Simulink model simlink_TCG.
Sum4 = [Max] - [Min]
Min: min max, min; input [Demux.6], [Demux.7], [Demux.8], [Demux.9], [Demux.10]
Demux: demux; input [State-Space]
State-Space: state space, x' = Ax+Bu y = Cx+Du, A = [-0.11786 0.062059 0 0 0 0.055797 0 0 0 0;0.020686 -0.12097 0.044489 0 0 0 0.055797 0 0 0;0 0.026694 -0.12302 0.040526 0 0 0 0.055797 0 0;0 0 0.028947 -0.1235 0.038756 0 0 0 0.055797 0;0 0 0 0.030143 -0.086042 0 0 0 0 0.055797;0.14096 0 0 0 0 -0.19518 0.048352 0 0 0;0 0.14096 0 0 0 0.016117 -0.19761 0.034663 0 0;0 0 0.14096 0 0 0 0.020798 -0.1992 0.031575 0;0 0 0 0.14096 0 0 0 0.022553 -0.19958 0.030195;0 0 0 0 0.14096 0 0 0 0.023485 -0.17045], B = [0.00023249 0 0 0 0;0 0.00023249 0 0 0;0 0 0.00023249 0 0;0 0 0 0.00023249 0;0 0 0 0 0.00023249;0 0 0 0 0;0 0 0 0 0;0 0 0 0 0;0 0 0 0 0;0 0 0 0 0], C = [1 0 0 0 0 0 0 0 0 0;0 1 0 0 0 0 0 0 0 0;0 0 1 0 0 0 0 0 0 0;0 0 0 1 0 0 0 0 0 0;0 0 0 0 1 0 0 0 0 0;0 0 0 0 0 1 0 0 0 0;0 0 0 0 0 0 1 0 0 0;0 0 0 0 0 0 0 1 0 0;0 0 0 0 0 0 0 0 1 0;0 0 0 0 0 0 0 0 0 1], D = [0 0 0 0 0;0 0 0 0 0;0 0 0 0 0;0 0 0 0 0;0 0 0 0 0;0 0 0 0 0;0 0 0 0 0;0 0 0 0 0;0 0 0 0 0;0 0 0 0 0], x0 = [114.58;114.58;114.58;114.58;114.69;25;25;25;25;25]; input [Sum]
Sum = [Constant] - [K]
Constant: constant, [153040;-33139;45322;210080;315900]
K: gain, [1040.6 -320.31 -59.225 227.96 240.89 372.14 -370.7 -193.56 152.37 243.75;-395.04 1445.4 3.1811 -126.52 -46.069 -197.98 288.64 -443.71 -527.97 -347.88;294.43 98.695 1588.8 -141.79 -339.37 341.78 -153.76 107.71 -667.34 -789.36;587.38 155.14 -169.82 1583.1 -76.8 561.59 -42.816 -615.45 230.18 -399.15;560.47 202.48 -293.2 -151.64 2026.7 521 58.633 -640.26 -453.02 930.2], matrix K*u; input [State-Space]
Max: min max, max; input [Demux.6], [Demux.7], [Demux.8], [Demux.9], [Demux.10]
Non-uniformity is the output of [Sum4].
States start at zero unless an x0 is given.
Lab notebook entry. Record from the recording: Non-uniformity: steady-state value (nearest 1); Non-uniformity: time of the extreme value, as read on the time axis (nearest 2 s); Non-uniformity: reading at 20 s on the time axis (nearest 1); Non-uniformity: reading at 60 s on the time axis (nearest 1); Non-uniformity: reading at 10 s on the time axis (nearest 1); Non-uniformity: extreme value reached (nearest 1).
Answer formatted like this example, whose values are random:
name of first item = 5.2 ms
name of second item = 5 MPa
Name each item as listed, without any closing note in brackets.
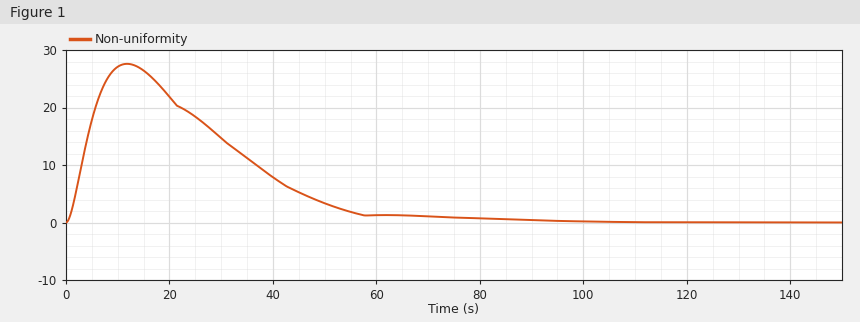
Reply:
Non-uniformity: steady-state value = 0
Non-uniformity: time of the extreme value, as read on the time axis = 12 s
Non-uniformity: reading at 20 s on the time axis = 22
Non-uniformity: reading at 60 s on the time axis = 1
Non-uniformity: reading at 10 s on the time axis = 27
Non-uniformity: extreme value reached = 28
